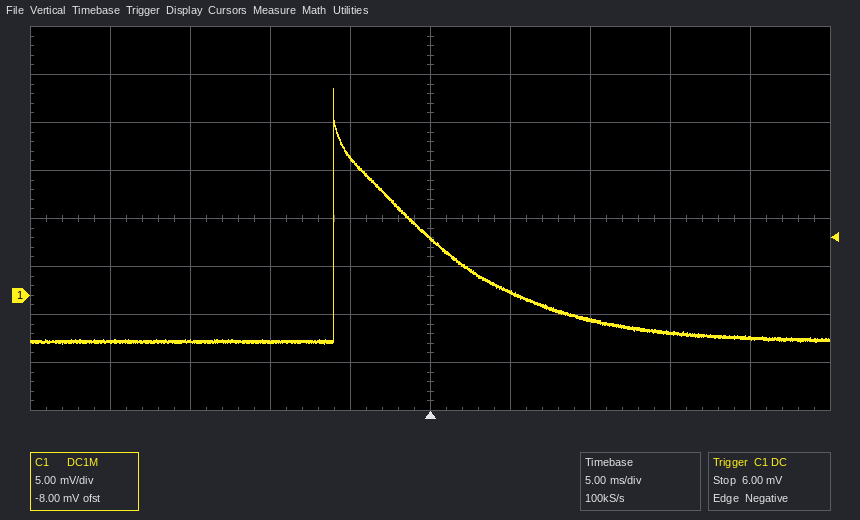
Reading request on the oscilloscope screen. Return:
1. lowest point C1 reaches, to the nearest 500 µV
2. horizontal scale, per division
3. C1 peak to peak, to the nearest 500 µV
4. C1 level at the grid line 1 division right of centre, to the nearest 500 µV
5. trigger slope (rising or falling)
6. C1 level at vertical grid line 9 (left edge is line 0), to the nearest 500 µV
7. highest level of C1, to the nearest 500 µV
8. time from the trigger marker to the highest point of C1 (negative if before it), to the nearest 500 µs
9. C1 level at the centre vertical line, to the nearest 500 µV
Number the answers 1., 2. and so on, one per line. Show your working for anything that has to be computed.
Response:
1. -5.0 mV
2. 5 ms
3. 21.5 mV − (-5.0 mV) = 26.5 mV
4. 500 µV
5. falling
6. -4.5 mV
7. 21.5 mV
8. -6.0 ms
9. 6.0 mV
